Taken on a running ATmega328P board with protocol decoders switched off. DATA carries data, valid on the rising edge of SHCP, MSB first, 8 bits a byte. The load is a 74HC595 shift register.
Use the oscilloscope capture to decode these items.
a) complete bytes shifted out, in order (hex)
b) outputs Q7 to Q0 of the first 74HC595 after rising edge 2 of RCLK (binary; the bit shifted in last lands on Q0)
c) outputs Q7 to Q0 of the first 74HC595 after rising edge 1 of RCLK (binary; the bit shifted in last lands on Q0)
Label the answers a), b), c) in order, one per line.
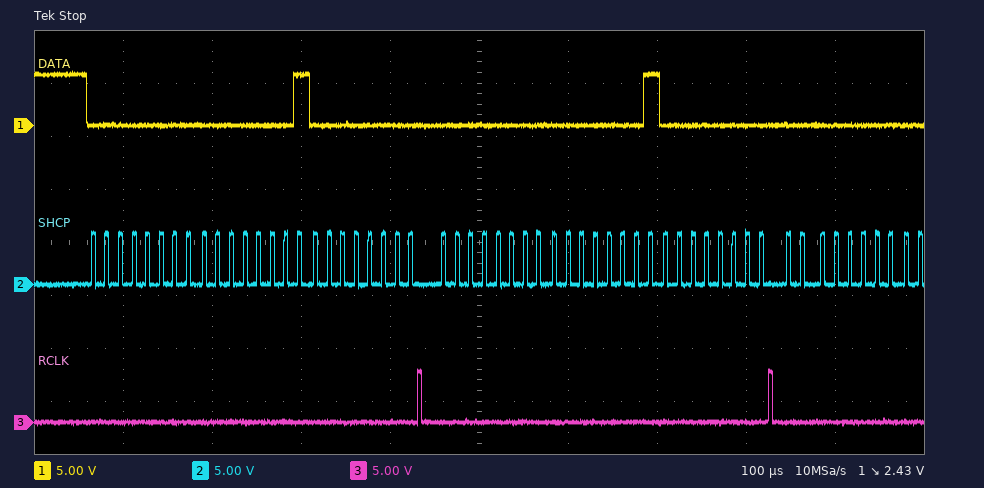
a) 00 01 00 00 01 00 00
b) 00000000
c) 00000000
